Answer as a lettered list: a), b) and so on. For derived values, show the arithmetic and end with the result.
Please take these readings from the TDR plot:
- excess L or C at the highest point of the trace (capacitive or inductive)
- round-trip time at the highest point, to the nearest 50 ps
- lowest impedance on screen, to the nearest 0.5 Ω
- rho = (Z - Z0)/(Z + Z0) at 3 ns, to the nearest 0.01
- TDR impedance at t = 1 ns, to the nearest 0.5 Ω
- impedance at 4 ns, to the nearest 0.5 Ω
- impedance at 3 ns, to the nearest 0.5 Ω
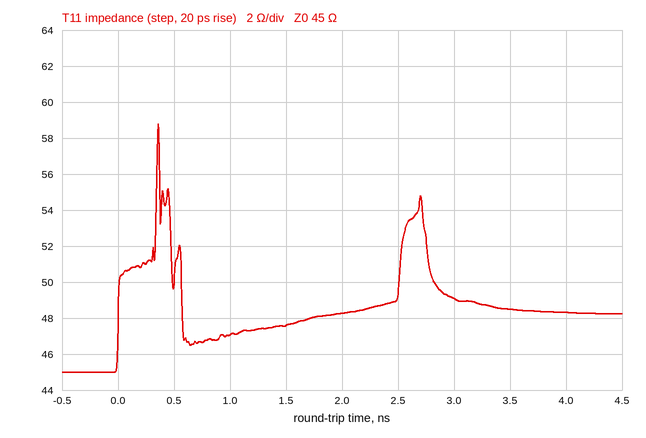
a) inductive
b) 350 ps
c) 45.0 Ω
d) (49 − 45)/(49 + 45) ≈ +0.04
e) 47.0 Ω
f) 48.5 Ω
g) 49.0 Ω
